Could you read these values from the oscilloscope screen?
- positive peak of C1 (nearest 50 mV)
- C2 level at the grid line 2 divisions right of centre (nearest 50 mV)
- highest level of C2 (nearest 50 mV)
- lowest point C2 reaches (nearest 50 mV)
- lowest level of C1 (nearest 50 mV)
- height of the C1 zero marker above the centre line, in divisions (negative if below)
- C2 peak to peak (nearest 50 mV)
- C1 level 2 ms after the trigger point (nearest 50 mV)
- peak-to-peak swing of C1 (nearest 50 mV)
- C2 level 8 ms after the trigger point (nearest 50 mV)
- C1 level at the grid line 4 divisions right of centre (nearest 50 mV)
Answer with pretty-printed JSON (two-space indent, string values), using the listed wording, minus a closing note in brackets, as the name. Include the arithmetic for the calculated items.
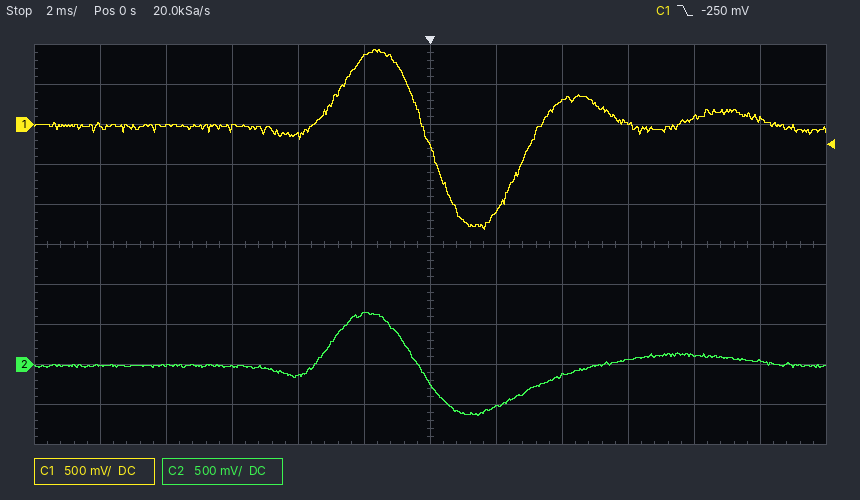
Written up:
{
  "positive peak of C1": "950 mV",
  "C2 level at the grid line 2 divisions right of centre": "-150 mV",
  "highest level of C2": "650 mV",
  "lowest point C2 reaches": "-650 mV",
  "lowest level of C1": "-1.30 V",
  "height of the C1 zero marker above the centre line, in divisions": "+3.0 div",
  "C2 peak to peak": "650 mV − (-650 mV) = 1.30 V",
  "C1 level 2 ms after the trigger point": "-1.10 V",
  "peak-to-peak swing of C1": "950 mV − (-1.30 V) = 2.25 V",
  "C2 level 8 ms after the trigger point": "100 mV",
  "C1 level at the grid line 4 divisions right of centre": "100 mV"
}
